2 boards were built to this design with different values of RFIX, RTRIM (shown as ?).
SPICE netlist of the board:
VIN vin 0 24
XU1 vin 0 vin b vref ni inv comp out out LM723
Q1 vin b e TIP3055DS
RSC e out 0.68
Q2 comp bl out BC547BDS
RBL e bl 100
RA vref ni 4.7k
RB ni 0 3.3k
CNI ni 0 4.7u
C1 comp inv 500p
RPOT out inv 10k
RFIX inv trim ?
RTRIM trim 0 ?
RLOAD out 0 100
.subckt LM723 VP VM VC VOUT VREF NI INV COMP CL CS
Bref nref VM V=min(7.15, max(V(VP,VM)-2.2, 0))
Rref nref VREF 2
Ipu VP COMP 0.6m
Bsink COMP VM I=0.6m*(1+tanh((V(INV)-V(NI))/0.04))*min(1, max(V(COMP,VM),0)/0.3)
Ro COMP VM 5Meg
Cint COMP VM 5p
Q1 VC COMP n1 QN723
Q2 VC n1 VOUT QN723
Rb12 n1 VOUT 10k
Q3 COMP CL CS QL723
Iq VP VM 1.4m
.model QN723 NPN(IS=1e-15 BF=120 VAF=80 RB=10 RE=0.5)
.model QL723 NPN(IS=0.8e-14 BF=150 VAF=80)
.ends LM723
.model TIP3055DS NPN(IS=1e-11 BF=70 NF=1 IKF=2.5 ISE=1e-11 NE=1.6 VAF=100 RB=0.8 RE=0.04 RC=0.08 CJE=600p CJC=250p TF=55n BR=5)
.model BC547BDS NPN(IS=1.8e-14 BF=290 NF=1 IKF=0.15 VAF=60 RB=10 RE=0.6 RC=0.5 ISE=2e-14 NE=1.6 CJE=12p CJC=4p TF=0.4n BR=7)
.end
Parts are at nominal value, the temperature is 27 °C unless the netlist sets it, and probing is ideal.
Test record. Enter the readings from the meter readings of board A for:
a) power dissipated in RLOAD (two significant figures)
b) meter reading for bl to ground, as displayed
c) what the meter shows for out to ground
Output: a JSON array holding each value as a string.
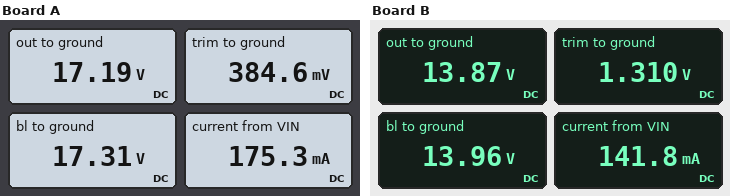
["3.0 W", "17.31 V", "17.19 V"]
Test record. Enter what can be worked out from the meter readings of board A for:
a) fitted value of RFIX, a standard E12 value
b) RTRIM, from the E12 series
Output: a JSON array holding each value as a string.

["1.8 kΩ", "270 Ω"]
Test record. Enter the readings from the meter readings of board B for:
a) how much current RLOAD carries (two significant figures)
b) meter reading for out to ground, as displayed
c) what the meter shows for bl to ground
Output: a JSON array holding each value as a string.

["140 mA", "13.87 V", "13.96 V"]
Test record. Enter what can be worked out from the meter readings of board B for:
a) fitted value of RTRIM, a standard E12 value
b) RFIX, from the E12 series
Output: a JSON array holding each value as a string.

["1.2 kΩ", "1.5 kΩ"]
